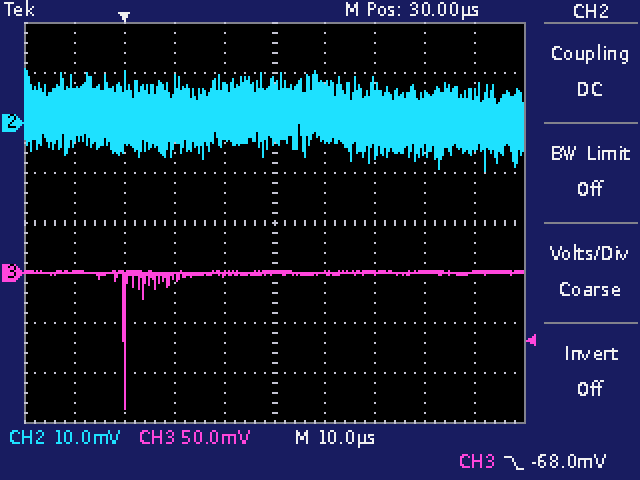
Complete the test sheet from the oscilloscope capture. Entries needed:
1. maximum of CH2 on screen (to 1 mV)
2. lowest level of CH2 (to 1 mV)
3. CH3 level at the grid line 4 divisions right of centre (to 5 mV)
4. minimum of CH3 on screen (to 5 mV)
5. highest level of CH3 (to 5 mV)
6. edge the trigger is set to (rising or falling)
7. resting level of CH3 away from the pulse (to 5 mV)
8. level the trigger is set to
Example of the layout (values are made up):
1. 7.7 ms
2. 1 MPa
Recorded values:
1. 11 mV
2. -10 mV
3. 0 mV
4. -135 mV
5. 0 mV
6. falling
7. 0 mV
8. -68.0 mV
